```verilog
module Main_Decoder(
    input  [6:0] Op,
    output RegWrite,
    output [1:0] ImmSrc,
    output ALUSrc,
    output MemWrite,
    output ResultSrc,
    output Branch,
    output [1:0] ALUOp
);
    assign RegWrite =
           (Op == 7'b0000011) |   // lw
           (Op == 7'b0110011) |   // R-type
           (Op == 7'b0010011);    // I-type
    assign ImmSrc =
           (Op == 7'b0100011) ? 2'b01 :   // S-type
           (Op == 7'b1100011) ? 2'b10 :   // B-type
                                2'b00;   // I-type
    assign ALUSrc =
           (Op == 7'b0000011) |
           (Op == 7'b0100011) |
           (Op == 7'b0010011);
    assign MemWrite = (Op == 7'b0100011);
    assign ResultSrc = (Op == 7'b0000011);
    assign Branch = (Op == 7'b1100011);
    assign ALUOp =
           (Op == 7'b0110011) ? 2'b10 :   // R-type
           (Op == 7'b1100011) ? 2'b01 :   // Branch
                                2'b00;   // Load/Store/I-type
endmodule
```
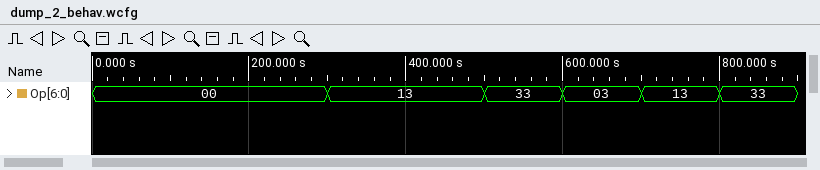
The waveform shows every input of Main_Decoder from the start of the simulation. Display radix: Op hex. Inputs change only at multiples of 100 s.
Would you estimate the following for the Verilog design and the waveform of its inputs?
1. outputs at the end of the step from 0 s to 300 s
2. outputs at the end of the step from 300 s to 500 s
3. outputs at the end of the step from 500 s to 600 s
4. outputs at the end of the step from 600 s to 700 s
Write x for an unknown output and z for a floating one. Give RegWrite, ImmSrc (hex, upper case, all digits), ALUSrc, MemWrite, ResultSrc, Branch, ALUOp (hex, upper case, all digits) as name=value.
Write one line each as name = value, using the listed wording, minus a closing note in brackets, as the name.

outputs at the end of the step from 0 s to 300 s = RegWrite=0, ImmSrc=0, ALUSrc=0, MemWrite=0, ResultSrc=0, Branch=0, ALUOp=0
outputs at the end of the step from 300 s to 500 s = RegWrite=1, ImmSrc=0, ALUSrc=1, MemWrite=0, ResultSrc=0, Branch=0, ALUOp=0
outputs at the end of the step from 500 s to 600 s = RegWrite=1, ImmSrc=0, ALUSrc=0, MemWrite=0, ResultSrc=0, Branch=0, ALUOp=2
outputs at the end of the step from 600 s to 700 s = RegWrite=1, ImmSrc=0, ALUSrc=1, MemWrite=0, ResultSrc=1, Branch=0, ALUOp=0
